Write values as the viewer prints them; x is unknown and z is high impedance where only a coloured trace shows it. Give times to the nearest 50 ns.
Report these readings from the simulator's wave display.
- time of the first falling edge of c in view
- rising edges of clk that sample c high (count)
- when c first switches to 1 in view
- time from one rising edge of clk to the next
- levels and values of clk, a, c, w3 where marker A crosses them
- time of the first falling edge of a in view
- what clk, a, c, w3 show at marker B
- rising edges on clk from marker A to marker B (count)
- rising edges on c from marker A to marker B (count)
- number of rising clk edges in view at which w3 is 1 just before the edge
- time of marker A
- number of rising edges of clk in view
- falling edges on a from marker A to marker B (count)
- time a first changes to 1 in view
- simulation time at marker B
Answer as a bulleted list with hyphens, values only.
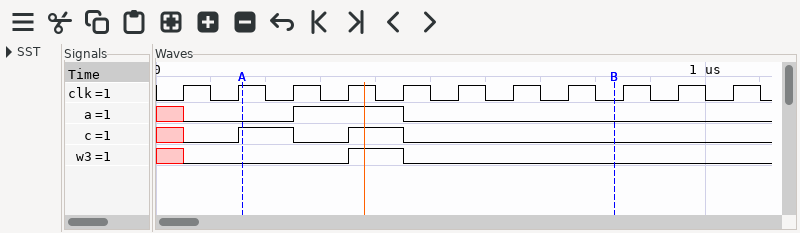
- 250 ns
- 2
- 150 ns
- 100 ns
- clk=1, a=0, c=1, w3=0
- 450 ns
- clk=0, a=0, c=0, w3=0
- 6
- 1
- 1
- 150 ns
- 11
- 1
- 250 ns
- 850 ns
